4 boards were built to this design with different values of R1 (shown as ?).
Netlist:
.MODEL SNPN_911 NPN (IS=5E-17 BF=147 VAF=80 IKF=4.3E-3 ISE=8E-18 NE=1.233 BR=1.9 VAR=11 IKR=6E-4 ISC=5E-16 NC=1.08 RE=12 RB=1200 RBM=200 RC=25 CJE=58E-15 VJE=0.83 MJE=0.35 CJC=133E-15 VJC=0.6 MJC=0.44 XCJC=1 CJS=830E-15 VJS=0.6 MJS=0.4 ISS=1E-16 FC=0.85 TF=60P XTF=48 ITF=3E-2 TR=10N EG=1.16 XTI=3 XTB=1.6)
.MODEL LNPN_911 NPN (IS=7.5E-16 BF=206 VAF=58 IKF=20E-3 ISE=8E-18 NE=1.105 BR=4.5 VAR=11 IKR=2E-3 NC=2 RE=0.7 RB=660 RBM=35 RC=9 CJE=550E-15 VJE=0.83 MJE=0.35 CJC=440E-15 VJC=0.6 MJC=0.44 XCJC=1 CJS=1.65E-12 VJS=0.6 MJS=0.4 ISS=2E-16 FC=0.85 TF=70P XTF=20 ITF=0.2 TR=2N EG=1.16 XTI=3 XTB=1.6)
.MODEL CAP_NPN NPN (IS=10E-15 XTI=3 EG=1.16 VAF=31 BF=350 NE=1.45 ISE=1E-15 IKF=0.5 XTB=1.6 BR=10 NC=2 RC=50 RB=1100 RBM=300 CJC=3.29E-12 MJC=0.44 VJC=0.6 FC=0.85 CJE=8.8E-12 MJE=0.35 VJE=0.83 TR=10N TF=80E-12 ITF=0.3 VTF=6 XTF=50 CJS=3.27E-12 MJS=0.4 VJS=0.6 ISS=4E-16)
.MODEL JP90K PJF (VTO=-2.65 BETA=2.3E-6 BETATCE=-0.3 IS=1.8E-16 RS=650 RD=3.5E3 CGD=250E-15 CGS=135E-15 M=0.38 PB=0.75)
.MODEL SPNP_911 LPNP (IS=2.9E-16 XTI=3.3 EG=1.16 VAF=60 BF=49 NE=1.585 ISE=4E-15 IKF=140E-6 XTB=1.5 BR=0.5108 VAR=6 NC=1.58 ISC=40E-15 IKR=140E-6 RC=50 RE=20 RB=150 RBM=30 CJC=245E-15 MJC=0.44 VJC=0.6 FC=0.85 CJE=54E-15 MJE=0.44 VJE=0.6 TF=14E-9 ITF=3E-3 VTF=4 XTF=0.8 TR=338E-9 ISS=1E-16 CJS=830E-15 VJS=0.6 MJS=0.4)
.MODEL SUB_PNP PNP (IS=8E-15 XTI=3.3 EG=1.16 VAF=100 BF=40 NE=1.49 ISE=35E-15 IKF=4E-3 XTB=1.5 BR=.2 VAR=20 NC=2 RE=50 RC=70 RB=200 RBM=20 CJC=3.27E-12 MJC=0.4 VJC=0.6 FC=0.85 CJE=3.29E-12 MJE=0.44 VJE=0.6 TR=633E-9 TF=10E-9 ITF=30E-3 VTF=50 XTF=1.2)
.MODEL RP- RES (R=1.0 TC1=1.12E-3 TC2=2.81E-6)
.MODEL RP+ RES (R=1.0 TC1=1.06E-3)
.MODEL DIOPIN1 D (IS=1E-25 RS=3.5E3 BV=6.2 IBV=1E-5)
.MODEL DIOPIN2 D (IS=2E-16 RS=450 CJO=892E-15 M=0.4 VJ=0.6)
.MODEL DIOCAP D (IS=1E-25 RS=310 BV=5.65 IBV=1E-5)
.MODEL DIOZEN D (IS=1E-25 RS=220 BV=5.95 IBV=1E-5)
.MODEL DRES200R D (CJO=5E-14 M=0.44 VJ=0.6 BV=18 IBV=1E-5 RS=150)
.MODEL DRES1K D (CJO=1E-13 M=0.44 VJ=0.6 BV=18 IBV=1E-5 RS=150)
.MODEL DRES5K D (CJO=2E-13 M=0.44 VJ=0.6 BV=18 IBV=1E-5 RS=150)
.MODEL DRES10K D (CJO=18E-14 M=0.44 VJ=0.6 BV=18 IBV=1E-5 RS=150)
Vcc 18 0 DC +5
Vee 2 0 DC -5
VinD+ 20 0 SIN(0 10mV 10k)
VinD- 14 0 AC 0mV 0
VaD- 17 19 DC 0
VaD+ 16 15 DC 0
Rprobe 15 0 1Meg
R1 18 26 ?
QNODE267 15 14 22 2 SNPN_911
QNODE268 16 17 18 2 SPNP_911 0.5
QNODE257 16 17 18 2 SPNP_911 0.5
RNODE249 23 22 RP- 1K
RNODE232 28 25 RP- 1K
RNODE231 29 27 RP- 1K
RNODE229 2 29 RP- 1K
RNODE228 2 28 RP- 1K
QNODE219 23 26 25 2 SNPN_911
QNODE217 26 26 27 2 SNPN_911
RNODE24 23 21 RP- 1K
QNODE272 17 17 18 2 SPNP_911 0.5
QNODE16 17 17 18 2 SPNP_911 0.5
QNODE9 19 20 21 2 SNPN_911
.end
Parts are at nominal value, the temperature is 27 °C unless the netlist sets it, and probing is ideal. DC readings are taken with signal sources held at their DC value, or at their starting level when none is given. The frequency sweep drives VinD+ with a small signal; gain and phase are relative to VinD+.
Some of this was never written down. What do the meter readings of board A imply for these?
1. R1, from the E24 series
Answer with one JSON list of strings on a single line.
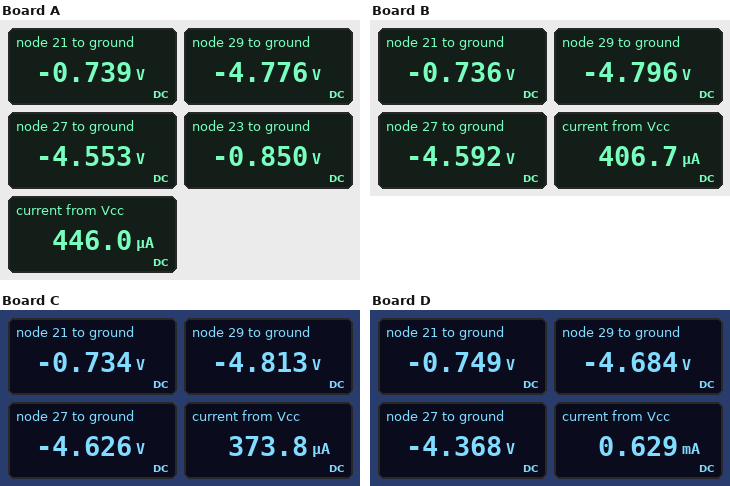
["39 kΩ"]
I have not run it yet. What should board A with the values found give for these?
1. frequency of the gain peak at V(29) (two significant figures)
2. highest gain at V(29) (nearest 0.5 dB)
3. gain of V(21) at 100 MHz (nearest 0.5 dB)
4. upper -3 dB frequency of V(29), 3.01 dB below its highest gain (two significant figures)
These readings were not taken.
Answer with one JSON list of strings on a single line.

["230 MHz", "-34.5 dB", "-1.0 dB", "550 MHz"]
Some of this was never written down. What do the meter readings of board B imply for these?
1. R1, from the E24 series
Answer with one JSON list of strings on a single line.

["43 kΩ"]
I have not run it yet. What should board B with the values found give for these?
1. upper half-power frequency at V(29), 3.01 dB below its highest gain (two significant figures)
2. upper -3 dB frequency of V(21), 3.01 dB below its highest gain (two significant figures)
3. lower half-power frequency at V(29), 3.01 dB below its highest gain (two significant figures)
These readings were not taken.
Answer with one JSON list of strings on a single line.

["540 MHz", "910 MHz", "82 MHz"]
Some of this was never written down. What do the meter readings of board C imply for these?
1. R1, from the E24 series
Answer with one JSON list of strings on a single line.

["47 kΩ"]
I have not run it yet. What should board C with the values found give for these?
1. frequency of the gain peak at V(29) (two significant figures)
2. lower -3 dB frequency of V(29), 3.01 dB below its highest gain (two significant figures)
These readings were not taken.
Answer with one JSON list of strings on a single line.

["220 MHz", "81 MHz"]
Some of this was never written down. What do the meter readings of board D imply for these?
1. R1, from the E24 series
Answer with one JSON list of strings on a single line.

["27 kΩ"]
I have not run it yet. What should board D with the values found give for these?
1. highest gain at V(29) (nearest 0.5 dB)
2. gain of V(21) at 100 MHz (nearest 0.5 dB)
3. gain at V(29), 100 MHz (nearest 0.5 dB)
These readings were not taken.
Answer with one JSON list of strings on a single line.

["-33.5 dB", "-0.5 dB", "-35.5 dB"]
